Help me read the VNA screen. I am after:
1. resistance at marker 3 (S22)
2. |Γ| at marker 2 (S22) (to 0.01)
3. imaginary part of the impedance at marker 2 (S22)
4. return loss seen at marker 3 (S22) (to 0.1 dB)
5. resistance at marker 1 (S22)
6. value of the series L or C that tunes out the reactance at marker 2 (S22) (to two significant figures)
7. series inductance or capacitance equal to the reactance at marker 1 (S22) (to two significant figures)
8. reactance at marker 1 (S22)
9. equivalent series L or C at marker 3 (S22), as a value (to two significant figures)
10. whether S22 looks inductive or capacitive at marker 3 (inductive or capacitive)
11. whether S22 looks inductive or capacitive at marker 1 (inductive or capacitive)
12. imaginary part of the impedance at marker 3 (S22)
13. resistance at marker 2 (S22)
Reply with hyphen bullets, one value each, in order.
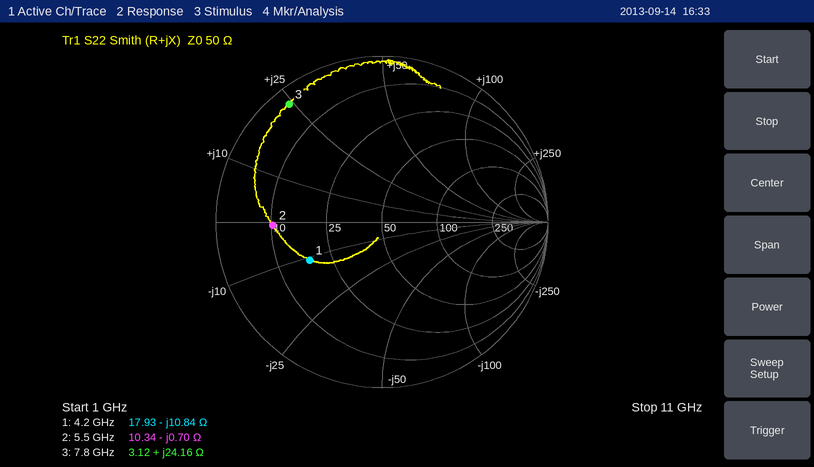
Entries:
- 3.12 Ω
- 0.66
- -0.70 Ω
- 0.9 dB
- 17.93 Ω
- 20 pH
- 3.5 pF
- -10.84 Ω
- 490 pH
- inductive
- capacitive
- +24.16 Ω
- 10.34 Ω
